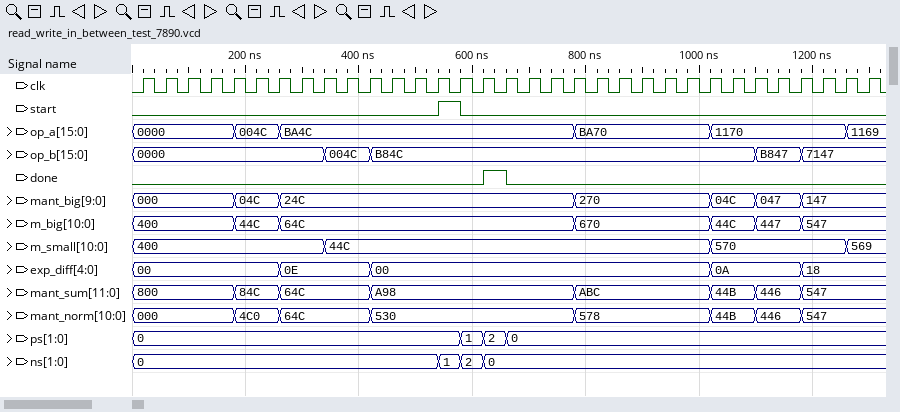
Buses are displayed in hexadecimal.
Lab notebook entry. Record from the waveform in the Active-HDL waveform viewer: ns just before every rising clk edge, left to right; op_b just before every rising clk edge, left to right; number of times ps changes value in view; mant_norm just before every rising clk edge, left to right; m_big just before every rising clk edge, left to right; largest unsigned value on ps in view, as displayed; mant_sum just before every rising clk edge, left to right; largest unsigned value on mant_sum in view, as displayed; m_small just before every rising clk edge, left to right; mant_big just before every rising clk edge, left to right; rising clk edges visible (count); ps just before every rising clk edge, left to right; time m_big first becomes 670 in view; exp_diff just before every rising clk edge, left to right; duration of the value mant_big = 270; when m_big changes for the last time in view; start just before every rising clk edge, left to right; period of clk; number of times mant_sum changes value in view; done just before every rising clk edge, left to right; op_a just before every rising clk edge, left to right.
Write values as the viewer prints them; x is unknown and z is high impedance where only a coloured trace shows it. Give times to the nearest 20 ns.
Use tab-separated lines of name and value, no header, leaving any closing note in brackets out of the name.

ns just before every rising clk edge, left to right	0, 0, 0, 0, 0, 0, 0, 0, 0, 0, 0, 0, 0, 0, 1, 2, 0, 0, 0, 0, 0, 0, 0, 0, 0, 0, 0, 0, 0, 0, 0, 0, 0
op_b just before every rising clk edge, left to right	0000, 0000, 0000, 0000, 0000, 0000, 0000, 0000, 0000, 004C, 004C, B84C, B84C, B84C, B84C, B84C, B84C, B84C, B84C, B84C, B84C, B84C, B84C, B84C, B84C, B84C, B84C, B84C, B847, B847, 7147, 7147, 7147
number of times ps changes value in view	3
mant_norm just before every rising clk edge, left to right	000, 000, 000, 000, 000, 4C0, 4C0, 64C, 64C, 64C, 64C, 530, 530, 530, 530, 530, 530, 530, 530, 530, 578, 578, 578, 578, 578, 578, 44B, 44B, 446, 446, 547, 547, 547
m_big just before every rising clk edge, left to right	400, 400, 400, 400, 400, 44C, 44C, 64C, 64C, 64C, 64C, 64C, 64C, 64C, 64C, 64C, 64C, 64C, 64C, 64C, 670, 670, 670, 670, 670, 670, 44C, 44C, 447, 447, 547, 547, 547
largest unsigned value on ps in view, as displayed	2
mant_sum just before every rising clk edge, left to right	800, 800, 800, 800, 800, 84C, 84C, 64C, 64C, 64C, 64C, A98, A98, A98, A98, A98, A98, A98, A98, A98, ABC, ABC, ABC, ABC, ABC, ABC, 44B, 44B, 446, 446, 547, 547, 547
largest unsigned value on mant_sum in view, as displayed	ABC
m_small just before every rising clk edge, left to right	400, 400, 400, 400, 400, 400, 400, 400, 400, 44C, 44C, 44C, 44C, 44C, 44C, 44C, 44C, 44C, 44C, 44C, 44C, 44C, 44C, 44C, 44C, 44C, 570, 570, 570, 570, 570, 570, 569
mant_big just before every rising clk edge, left to right	000, 000, 000, 000, 000, 04C, 04C, 24C, 24C, 24C, 24C, 24C, 24C, 24C, 24C, 24C, 24C, 24C, 24C, 24C, 270, 270, 270, 270, 270, 270, 04C, 04C, 047, 047, 147, 147, 147
rising clk edges visible	33
ps just before every rising clk edge, left to right	0, 0, 0, 0, 0, 0, 0, 0, 0, 0, 0, 0, 0, 0, 0, 1, 2, 0, 0, 0, 0, 0, 0, 0, 0, 0, 0, 0, 0, 0, 0, 0, 0
time m_big first becomes 670 in view	780 ns
exp_diff just before every rising clk edge, left to right	00, 00, 00, 00, 00, 00, 00, 0E, 0E, 0E, 0E, 00, 00, 00, 00, 00, 00, 00, 00, 00, 00, 00, 00, 00, 00, 00, 0A, 0A, 0A, 0A, 18, 18, 18
duration of the value mant_big = 270	240 ns
when m_big changes for the last time in view	1180 ns
start just before every rising clk edge, left to right	0 0 0 0 0 0 0 0 0 0 0 0 0 0 1 0 0 0 0 0 0 0 0 0 0 0 0 0 0 0 0 0 0
period of clk	40 ns
number of times mant_sum changes value in view	7
done just before every rising clk edge, left to right	0 0 0 0 0 0 0 0 0 0 0 0 0 0 0 0 1 0 0 0 0 0 0 0 0 0 0 0 0 0 0 0 0
op_a just before every rising clk edge, left to right	0000, 0000, 0000, 0000, 0000, 004C, 004C, BA4C, BA4C, BA4C, BA4C, BA4C, BA4C, BA4C, BA4C, BA4C, BA4C, BA4C, BA4C, BA4C, BA70, BA70, BA70, BA70, BA70, BA70, 1170, 1170, 1170, 1170, 1170, 1170, 1169
